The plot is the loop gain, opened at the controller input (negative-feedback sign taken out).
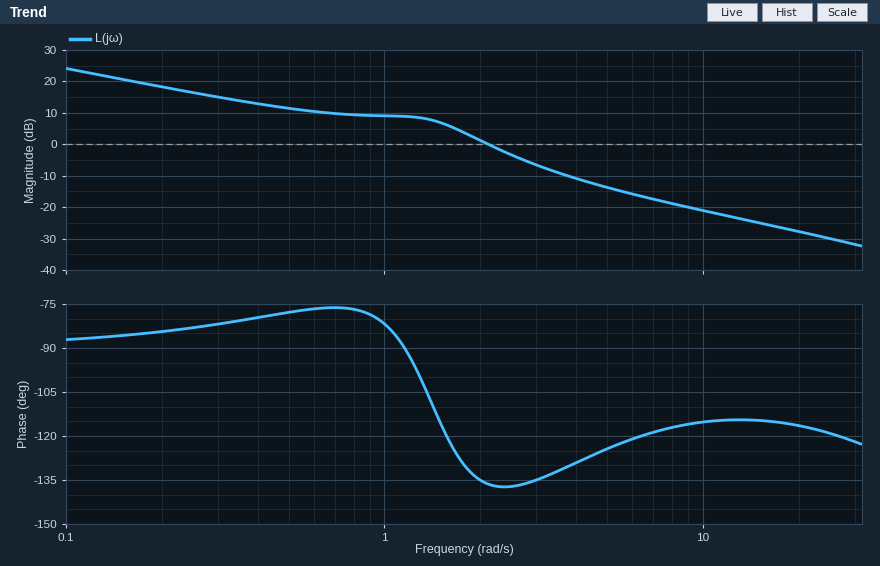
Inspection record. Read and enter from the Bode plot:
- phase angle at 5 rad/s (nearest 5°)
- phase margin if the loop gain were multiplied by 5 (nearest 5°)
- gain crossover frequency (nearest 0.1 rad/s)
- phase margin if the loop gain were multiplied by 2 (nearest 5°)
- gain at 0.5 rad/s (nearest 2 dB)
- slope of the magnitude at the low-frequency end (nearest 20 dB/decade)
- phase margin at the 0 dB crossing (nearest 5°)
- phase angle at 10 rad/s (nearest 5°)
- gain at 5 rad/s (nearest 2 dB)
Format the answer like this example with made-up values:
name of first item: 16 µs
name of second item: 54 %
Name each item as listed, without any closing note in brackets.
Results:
phase angle at 5 rad/s: -125°
phase margin if the loop gain were multiplied by 5: 55°
gain crossover frequency: 2.1 rad/s
phase margin if the loop gain were multiplied by 2: 45°
gain at 0.5 rad/s: 12 dB
slope of the magnitude at the low-frequency end: -20 dB/decade
phase margin at the 0 dB crossing: 45°
phase angle at 10 rad/s: -115°
gain at 5 rad/s: -14 dB
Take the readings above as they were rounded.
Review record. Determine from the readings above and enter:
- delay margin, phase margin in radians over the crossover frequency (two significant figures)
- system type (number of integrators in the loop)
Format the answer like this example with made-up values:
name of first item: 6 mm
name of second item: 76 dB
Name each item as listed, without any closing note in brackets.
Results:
delay margin, phase margin in radians over the crossover frequency: 0.37 s
system type: 1
